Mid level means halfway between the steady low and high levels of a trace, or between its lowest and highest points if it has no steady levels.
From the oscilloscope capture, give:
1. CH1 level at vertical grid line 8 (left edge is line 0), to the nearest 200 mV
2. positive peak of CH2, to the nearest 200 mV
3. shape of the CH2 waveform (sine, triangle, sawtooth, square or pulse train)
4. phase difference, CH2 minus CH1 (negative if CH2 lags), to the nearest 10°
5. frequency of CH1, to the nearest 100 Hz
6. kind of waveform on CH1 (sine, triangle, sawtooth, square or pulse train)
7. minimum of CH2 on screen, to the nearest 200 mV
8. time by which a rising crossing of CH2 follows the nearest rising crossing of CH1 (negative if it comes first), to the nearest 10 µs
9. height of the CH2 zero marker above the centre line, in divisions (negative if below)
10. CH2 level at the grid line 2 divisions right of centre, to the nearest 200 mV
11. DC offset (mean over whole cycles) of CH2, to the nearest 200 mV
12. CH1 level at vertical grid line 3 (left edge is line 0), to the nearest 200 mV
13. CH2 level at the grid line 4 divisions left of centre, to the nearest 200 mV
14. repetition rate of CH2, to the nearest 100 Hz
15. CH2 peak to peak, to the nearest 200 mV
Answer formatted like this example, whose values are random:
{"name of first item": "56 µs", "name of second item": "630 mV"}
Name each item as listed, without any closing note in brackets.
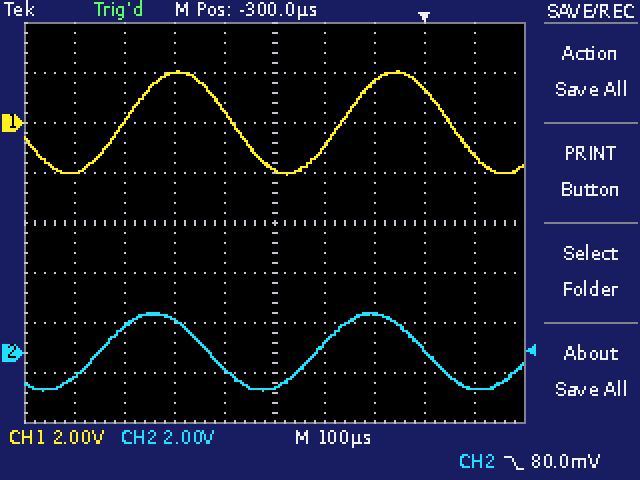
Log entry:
{"CH1 level at vertical grid line 8 (left edge is line 0), to the nearest 200 mV": "1.4 V", "positive peak of CH2, to the nearest 200 mV": "1.6 V", "shape of the CH2 waveform": "sine", "phase difference, CH2 minus CH1 (negative if CH2 lags), to the nearest 10°": "+40°", "frequency of CH1, to the nearest 100 Hz": "2.3 kHz", "kind of waveform on CH1": "sine", "minimum of CH2 on screen, to the nearest 200 mV": "-1.6 V", "time by which a rising crossing of CH2 follows the nearest rising crossing of CH1 (negative if it comes first), to the nearest 10 µs": "-50 µs", "height of the CH2 zero marker above the centre line, in divisions": "-2.6 div", "CH2 level at the grid line 2 divisions right of centre, to the nearest 200 mV": "1.6 V", "DC offset (mean over whole cycles) of CH2, to the nearest 200 mV": "0.0 V", "CH1 level at vertical grid line 3 (left edge is line 0), to the nearest 200 mV": "2.0 V", "CH2 level at the grid line 4 divisions left of centre, to the nearest 200 mV": "-1.0 V", "repetition rate of CH2, to the nearest 100 Hz": "2.3 kHz", "CH2 peak to peak, to the nearest 200 mV": "3.2 V"}
